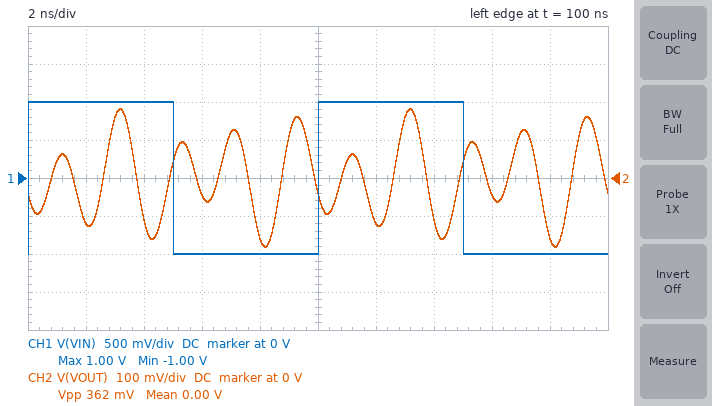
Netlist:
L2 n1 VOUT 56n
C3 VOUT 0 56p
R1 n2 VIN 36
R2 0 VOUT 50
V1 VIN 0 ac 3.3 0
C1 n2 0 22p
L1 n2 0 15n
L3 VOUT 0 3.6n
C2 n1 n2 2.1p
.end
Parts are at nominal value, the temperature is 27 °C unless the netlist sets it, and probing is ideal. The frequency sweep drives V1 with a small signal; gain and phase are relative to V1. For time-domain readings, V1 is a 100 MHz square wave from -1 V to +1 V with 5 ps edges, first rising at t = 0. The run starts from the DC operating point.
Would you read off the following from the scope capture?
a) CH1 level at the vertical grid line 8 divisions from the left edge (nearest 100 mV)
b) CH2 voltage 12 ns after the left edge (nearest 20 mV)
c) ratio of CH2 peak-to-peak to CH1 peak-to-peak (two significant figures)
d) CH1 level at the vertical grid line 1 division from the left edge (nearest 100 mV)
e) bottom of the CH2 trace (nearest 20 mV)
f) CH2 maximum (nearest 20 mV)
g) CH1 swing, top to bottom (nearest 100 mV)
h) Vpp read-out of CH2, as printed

-1.0 V
-120 mV
0.18
1.0 V
-180 mV
180 mV
2.0 V
362 mV
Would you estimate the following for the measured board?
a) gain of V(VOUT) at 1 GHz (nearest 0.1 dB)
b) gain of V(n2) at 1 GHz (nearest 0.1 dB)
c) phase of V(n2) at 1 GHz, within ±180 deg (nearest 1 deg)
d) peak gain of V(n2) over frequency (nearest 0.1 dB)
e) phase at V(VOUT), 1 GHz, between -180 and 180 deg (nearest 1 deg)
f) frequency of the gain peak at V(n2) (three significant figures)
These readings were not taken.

-51.7 dB
-13.2 dB
-77 deg
0 dB
106 deg
258 MHz
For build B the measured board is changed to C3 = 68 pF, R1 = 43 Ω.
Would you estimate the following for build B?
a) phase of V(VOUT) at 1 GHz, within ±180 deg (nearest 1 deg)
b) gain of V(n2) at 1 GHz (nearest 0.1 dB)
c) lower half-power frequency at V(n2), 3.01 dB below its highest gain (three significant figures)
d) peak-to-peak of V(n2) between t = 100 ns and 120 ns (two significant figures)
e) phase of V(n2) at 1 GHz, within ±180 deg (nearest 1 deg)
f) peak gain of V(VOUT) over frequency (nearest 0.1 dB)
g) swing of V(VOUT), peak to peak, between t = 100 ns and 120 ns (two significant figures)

104 deg
-14.7 dB
197 MHz
1.5 V
-79 deg
-8.8 dB
380 mV
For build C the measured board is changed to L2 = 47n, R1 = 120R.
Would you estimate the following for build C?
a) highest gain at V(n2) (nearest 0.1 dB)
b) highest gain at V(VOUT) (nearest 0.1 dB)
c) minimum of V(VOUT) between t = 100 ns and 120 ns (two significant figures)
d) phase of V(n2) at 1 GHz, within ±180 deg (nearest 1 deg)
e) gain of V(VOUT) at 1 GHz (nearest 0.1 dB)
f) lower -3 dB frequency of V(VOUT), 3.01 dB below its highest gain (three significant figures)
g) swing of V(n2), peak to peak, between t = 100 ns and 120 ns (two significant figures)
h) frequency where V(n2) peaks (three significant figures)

-0.1 dB
-10.1 dB
-45 mV
-86 deg
-59.9 dB
545 MHz
610 mV
260 MHz
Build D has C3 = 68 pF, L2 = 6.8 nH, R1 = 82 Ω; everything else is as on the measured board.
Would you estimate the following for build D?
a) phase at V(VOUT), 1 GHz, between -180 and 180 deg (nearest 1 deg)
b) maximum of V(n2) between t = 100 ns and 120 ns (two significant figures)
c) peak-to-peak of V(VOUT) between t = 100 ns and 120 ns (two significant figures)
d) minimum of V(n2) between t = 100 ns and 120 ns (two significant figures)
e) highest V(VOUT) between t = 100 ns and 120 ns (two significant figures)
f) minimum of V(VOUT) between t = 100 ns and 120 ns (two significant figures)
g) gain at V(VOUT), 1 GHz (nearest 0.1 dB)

-83 deg
490 mV
110 mV
-490 mV
56 mV
-56 mV
-44.9 dB
